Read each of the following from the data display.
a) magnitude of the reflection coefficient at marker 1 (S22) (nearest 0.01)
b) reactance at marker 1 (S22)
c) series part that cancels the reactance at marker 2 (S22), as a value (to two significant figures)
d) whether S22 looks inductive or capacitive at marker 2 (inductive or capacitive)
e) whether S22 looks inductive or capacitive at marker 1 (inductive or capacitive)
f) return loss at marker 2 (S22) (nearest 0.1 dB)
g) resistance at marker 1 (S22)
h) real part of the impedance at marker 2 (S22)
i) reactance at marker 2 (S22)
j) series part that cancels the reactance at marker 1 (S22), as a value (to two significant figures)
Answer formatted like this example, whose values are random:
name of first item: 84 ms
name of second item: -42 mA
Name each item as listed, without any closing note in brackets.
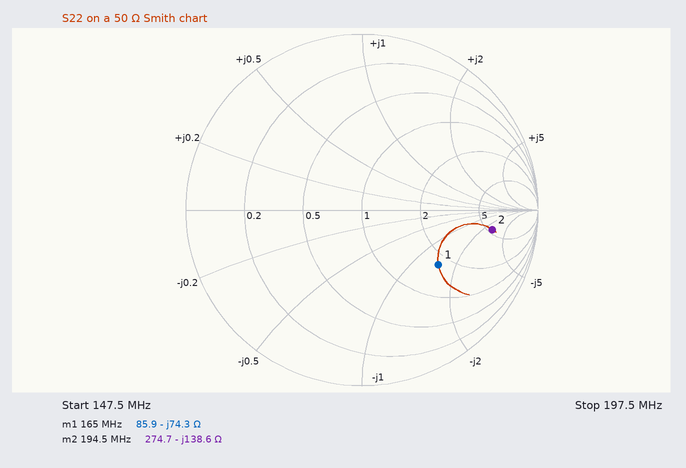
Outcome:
magnitude of the reflection coefficient at marker 1 (S22): 0.53
reactance at marker 1: -74.3 Ω
series part that cancels the reactance at marker 2 (S22), as a value: 110 nH
whether S22 looks inductive or capacitive at marker 2: capacitive
whether S22 looks inductive or capacitive at marker 1: capacitive
return loss at marker 2 (S22): 2.5 dB
resistance at marker 1: 85.9 Ω
real part of the impedance at marker 2: 274.7 Ω
reactance at marker 2: -138.6 Ω
series part that cancels the reactance at marker 1 (S22), as a value: 72 nH
